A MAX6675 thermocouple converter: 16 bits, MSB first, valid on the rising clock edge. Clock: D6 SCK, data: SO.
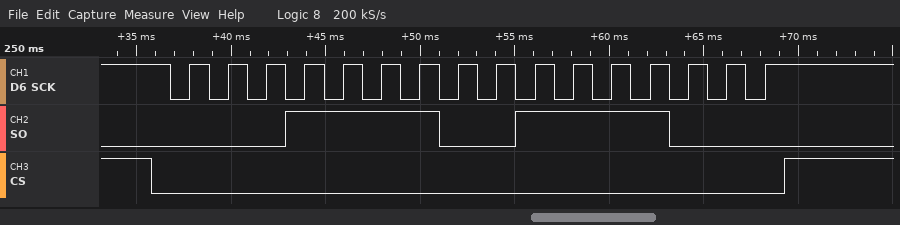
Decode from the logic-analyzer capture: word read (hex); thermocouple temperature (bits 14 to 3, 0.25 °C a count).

0x1E78
243.75 °C
